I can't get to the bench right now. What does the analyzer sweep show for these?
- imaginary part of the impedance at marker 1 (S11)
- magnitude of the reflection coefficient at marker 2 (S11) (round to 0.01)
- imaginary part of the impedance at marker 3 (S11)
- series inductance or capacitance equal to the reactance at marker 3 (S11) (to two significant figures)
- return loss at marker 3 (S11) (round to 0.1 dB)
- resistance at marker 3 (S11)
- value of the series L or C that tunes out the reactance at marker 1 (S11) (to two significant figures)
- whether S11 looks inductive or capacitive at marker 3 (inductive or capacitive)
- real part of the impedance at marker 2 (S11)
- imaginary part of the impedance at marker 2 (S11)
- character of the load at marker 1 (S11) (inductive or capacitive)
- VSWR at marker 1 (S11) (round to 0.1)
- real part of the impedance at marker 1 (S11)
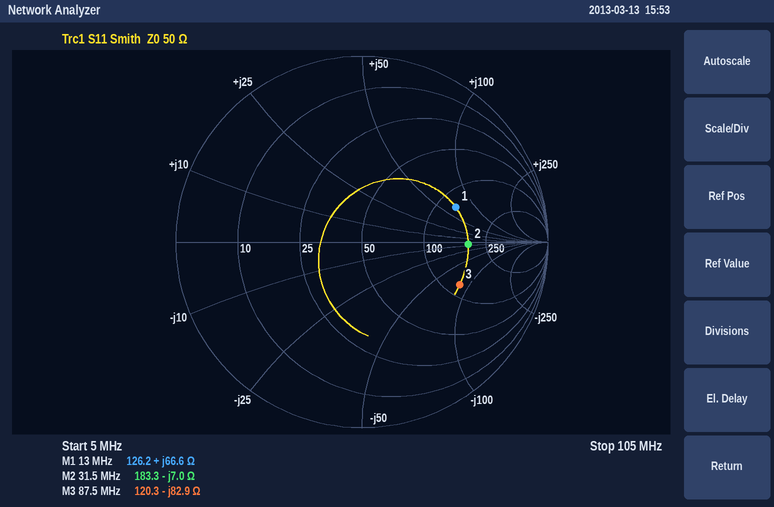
+66.6 Ω
0.57
-82.9 Ω
22 pF
4.8 dB
120.3 Ω
180 pF
capacitive
183.3 Ω
-7.0 Ω
inductive
3.3
126.2 Ω
